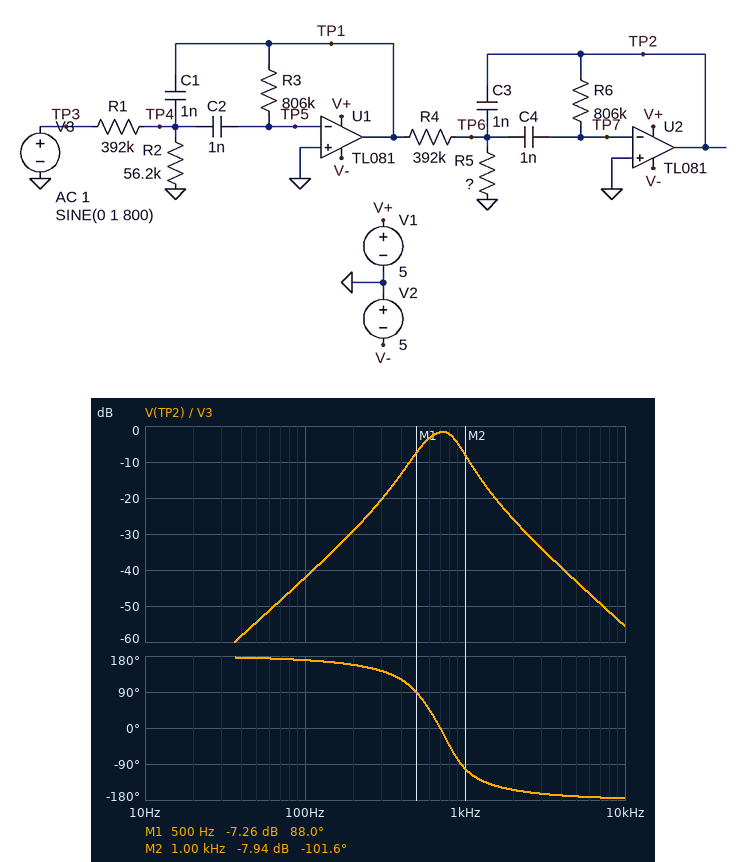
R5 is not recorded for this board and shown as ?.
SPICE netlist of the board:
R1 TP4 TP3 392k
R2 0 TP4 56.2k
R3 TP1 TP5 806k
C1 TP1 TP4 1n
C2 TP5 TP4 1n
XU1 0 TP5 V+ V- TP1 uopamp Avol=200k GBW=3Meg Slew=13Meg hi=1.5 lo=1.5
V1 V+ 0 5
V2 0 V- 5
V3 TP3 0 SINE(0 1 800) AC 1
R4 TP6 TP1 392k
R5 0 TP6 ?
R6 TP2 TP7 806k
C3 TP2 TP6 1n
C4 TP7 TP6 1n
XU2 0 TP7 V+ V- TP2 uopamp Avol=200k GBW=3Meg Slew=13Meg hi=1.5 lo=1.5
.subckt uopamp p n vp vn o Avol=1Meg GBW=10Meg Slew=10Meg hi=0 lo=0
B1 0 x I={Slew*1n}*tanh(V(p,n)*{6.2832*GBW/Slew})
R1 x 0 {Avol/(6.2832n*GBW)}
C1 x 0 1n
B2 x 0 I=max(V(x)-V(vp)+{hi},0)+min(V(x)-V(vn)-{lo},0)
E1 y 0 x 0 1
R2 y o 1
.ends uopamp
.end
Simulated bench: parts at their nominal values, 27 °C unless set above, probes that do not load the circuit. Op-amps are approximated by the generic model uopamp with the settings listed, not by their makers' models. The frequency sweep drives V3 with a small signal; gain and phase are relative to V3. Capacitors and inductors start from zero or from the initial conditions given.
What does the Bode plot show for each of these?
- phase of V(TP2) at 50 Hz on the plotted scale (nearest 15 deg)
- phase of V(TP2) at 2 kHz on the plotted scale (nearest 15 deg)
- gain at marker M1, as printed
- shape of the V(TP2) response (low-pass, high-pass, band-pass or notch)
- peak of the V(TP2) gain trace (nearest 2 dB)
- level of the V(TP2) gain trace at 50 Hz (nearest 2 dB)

180 deg
-150 deg
-7.26 dB
band-pass
-2 dB
-54 dB
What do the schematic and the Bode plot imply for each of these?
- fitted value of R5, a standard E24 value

120 kΩ
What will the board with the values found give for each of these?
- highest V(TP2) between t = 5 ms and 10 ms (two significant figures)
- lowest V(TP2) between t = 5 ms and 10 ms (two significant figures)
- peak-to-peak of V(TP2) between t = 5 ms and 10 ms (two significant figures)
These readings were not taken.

770 mV
-770 mV
1.5 V
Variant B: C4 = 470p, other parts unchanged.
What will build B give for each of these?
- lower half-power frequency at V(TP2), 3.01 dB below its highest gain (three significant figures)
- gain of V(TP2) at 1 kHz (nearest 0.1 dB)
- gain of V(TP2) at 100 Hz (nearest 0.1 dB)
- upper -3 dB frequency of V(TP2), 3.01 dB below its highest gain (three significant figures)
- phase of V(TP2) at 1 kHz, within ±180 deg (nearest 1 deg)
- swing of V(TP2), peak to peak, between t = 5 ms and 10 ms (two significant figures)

678 Hz
-6.8 dB
-48.8 dB
988 Hz
-66 deg
1.3 V
